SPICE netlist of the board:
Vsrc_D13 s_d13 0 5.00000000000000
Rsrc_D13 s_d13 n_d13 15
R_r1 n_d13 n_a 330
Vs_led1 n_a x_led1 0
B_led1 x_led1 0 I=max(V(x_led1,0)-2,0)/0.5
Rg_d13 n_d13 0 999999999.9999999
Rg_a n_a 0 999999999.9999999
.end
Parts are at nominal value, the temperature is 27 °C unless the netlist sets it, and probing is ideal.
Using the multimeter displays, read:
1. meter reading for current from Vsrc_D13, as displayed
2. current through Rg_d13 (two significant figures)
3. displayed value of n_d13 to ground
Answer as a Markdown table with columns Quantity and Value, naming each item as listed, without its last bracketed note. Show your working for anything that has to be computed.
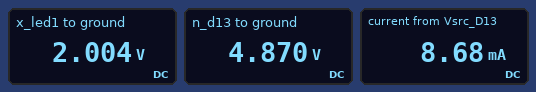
| Quantity | Value |
|---|---|
| meter reading for current from Vsrc_D13, as displayed | 8.68 mA |
| current through Rg_d13 | (4.87 V) / 1 GΩ = 4.9 nA |
| displayed value of n_d13 to ground | 4.870 V |
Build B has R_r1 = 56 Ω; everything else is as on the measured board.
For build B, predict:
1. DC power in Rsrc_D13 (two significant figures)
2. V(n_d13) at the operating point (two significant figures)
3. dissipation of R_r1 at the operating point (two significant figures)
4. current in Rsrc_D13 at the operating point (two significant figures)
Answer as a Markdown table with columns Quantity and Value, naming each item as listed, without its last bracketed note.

| Quantity | Value |
|---|---|
| DC power in Rsrc_D13 | 26 mW |
| V(n_d13) at the operating point | 4.4 V |
| dissipation of R_r1 at the operating point | 99 mW |
| current in Rsrc_D13 at the operating point | 42 mA |
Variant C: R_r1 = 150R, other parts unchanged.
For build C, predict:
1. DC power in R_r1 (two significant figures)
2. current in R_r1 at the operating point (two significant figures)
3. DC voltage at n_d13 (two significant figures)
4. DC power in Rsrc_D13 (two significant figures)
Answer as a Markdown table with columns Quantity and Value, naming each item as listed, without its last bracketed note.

| Quantity | Value |
|---|---|
| DC power in R_r1 | 49 mW |
| current in R_r1 at the operating point | 18 mA |
| DC voltage at n_d13 | 4.7 V |
| DC power in Rsrc_D13 | 4.9 mW |
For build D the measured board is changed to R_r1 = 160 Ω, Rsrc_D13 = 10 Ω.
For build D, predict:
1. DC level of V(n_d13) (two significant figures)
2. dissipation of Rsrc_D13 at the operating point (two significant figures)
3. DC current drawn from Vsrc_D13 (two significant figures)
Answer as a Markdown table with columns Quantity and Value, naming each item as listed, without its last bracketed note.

| Quantity | Value |
|---|---|
| DC level of V(n_d13) | 4.8 V |
| dissipation of Rsrc_D13 at the operating point | 3.1 mW |
| DC current drawn from Vsrc_D13 | 18 mA |
